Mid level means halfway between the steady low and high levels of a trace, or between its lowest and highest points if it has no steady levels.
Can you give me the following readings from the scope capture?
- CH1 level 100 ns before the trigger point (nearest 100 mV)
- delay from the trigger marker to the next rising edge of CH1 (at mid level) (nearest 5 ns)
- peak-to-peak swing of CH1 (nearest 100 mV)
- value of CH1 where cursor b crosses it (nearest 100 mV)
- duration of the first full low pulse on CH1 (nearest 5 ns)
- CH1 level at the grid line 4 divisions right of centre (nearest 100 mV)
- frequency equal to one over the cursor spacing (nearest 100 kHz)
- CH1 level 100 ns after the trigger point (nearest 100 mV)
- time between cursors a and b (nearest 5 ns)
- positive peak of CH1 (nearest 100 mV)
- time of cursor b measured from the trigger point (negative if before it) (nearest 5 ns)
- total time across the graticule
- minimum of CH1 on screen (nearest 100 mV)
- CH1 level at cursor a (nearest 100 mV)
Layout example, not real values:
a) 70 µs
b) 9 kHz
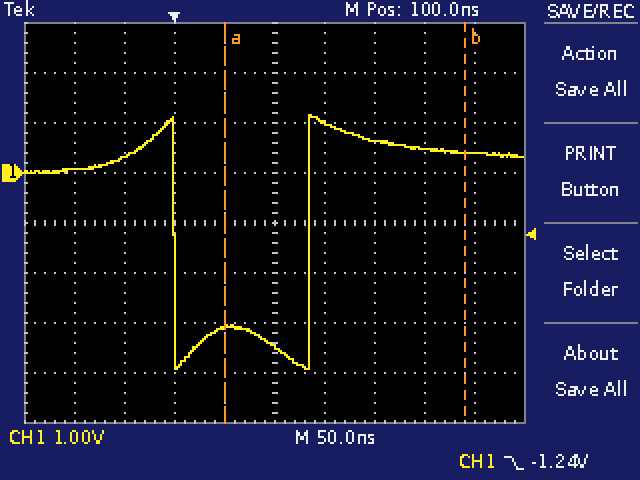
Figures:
a) 100 mV
b) 135 ns
c) 5.1 V
d) 400 mV
e) 135 ns
f) 400 mV
g) 4.2 MHz
h) -3.5 V
i) 240 ns
j) 1.2 V
k) +290 ns
l) 500 ns
m) -3.9 V
n) -3.1 V
